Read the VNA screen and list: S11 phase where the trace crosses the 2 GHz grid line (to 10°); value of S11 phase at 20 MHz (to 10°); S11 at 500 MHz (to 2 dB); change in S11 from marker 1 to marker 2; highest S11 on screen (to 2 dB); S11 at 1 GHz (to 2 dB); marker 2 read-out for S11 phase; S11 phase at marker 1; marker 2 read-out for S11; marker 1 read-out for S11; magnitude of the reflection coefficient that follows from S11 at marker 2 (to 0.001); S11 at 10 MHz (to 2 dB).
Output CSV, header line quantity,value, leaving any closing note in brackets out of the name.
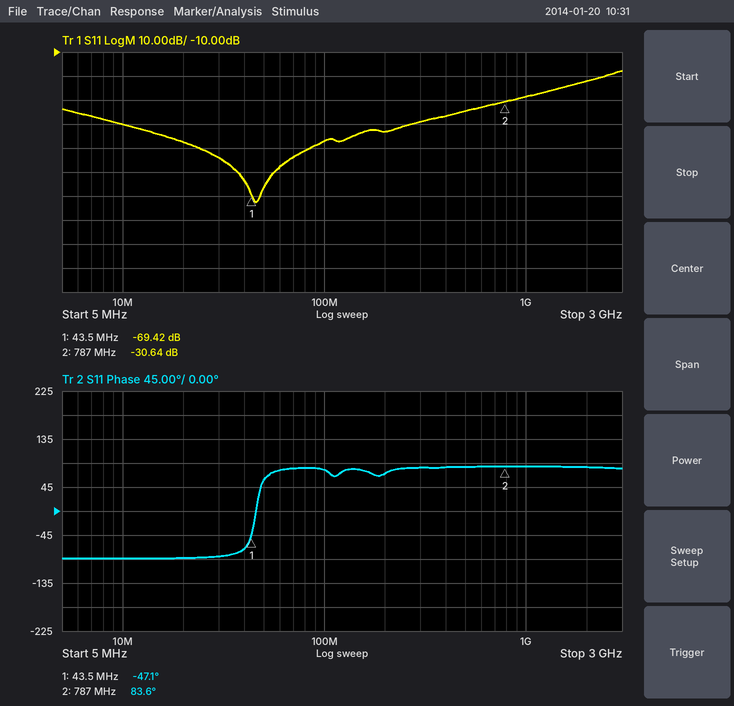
quantity,value
S11 phase where the trace crosses the 2 GHz grid line,80°
value of S11 phase at 20 MHz,-90°
S11 at 500 MHz,-34 dB
change in S11 from marker 1 to marker 2,38.78 dB
highest S11 on screen,-18 dB
S11 at 1 GHz,-28 dB
marker 2 read-out for S11 phase,83.6°
S11 phase at marker 1,-47.1°
marker 2 read-out for S11,-30.64 dB
marker 1 read-out for S11,-69.42 dB
magnitude of the reflection coefficient that follows from S11 at marker 2,0.029
S11 at 10 MHz,-40 dB
